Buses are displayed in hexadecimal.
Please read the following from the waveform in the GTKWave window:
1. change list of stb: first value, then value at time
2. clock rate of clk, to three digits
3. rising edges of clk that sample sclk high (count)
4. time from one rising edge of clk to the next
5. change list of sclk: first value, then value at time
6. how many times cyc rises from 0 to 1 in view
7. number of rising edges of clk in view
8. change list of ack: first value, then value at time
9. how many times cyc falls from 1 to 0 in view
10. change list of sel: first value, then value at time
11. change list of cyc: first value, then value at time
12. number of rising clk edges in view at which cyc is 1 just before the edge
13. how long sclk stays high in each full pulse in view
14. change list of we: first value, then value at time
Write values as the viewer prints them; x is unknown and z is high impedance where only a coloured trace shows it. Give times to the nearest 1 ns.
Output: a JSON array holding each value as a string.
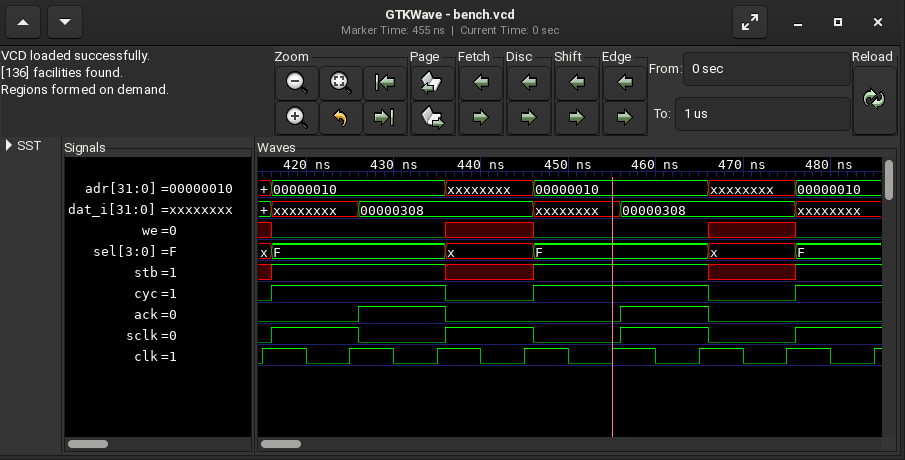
["x, 1 at 416 ns, x at 436 ns, 1 at 446 ns, x at 466 ns, 1 at 476 ns", "100 MHz", "4", "10 ns", "0, 1 at 416 ns, 0 at 426 ns, 1 at 436 ns, 0 at 446 ns, 1 at 456 ns, 0 at 466 ns, 1 at 476 ns", "3", "8", "0, 1 at 426 ns, 0 at 436 ns, 1 at 456 ns, 0 at 466 ns", "2", "x, F at 416 ns, x at 436 ns, F at 446 ns, x at 466 ns, F at 476 ns", "0, 1 at 416 ns, 0 at 436 ns, 1 at 446 ns, 0 at 466 ns, 1 at 476 ns", "5", "10 ns, 10 ns, 10 ns", "x, 0 at 416 ns, x at 436 ns, 0 at 446 ns, x at 466 ns, 0 at 476 ns"]
